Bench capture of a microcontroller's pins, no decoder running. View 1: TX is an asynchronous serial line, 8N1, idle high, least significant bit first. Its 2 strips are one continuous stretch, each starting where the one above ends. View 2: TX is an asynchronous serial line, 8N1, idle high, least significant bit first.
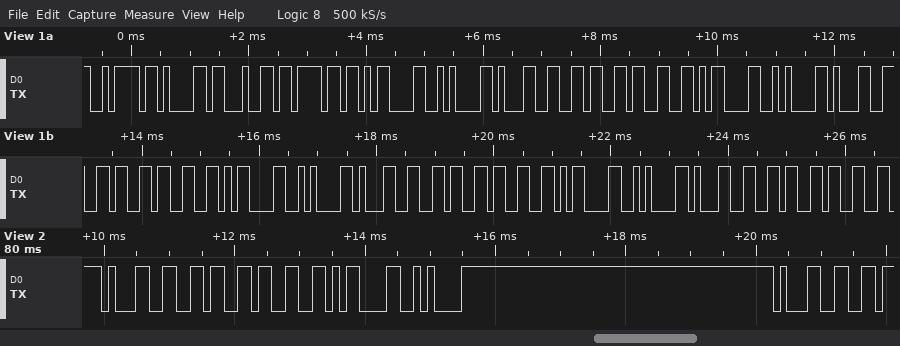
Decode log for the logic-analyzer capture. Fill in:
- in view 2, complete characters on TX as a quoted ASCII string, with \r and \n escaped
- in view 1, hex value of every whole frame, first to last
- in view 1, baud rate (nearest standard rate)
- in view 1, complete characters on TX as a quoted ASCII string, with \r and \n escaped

"163\r\n1"
7A 61 64 6F 0D 0A 31 36 33 0D 0A 31 36 33 0D 0A 31 36 33 0D 0A 31 36 33
9600 baud
"zado\r\n163\r\n163\r\n163\r\n163"
